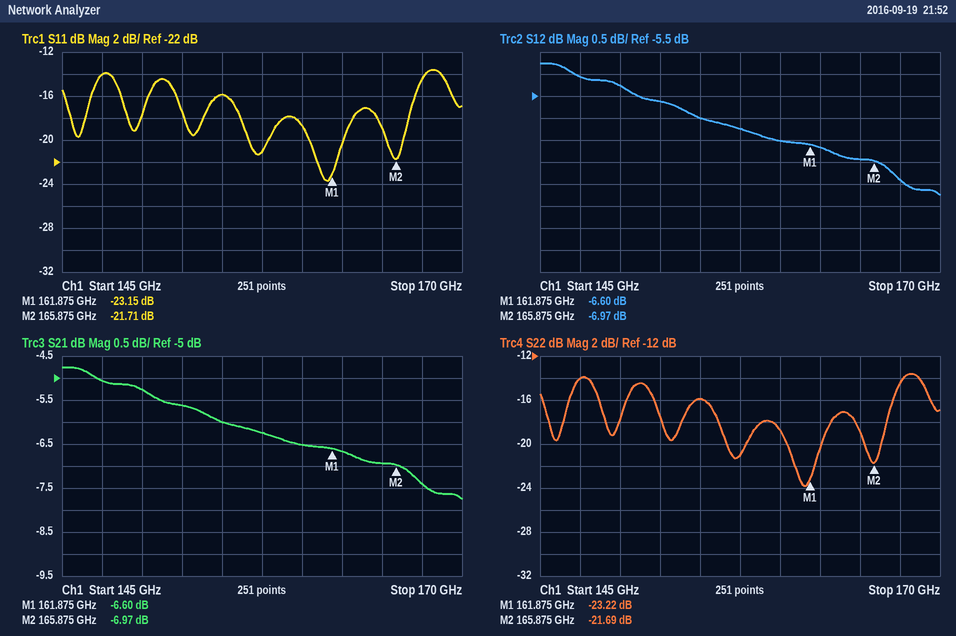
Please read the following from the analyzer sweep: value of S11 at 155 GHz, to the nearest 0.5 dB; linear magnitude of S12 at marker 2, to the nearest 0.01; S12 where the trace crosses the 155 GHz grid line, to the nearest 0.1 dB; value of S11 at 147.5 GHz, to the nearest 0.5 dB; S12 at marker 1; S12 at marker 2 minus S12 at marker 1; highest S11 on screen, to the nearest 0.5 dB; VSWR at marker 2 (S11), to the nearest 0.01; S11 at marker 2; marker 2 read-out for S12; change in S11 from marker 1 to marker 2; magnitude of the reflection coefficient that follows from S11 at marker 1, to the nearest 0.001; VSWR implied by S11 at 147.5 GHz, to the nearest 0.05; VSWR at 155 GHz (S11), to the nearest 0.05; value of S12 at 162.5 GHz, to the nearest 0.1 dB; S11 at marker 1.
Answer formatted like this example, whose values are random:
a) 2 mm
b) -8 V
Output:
a) -16.0 dB
b) 0.45
c) -6.0 dB
d) -14.0 dB
e) -6.60 dB
f) -0.37 dB
g) -13.5 dB
h) 1.18
i) -21.71 dB
j) -6.97 dB
k) 1.44 dB
l) 0.070
m) 1.50
n) 1.40
o) -6.7 dB
p) -23.15 dB
